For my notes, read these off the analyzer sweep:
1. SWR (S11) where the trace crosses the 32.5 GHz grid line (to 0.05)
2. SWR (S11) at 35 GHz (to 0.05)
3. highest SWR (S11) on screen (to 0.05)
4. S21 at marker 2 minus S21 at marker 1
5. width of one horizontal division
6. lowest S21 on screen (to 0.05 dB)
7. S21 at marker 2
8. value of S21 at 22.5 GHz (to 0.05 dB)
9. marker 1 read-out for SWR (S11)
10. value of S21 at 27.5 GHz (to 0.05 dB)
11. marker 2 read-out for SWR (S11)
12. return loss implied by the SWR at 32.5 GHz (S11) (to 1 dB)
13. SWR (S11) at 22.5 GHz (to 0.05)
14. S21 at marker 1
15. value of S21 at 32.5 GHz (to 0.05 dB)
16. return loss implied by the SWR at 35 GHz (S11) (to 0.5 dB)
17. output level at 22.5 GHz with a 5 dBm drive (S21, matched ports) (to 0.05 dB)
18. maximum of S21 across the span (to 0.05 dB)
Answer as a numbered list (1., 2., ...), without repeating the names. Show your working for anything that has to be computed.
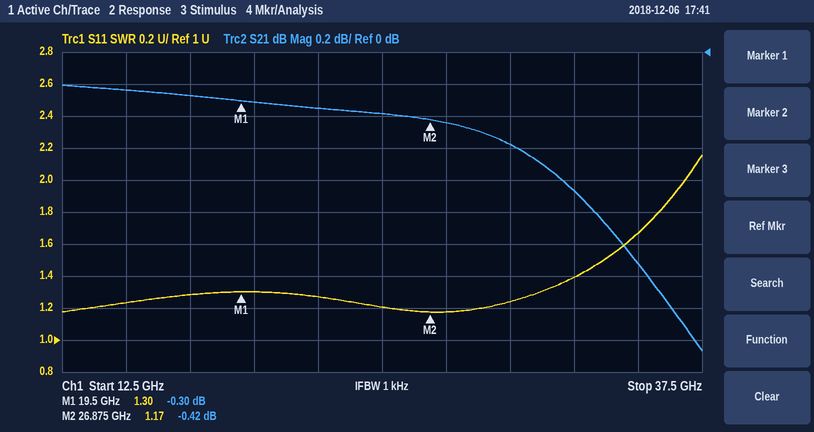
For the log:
1. 1.40
2. 1.65
3. 2.15
4. -0.42 − (-0.3) = -0.12 dB
5. 2.5 GHz
6. -1.85 dB
7. -0.42 dB
8. -0.35 dB
9. 1.30
10. -0.45 dB
11. 1.17
12. −20 log10((1.4 − 1)/(1.4 + 1)) ≈ 16 dB
13. 1.25
14. -0.30 dB
15. -0.85 dB
16. −20 log10((1.65 − 1)/(1.65 + 1)) ≈ 12.2 dB, so 12.0 dB to the nearest 0.5 dB
17. 5 dBm + (-0.35 dB) = 4.65 dBm
18. -0.20 dB
